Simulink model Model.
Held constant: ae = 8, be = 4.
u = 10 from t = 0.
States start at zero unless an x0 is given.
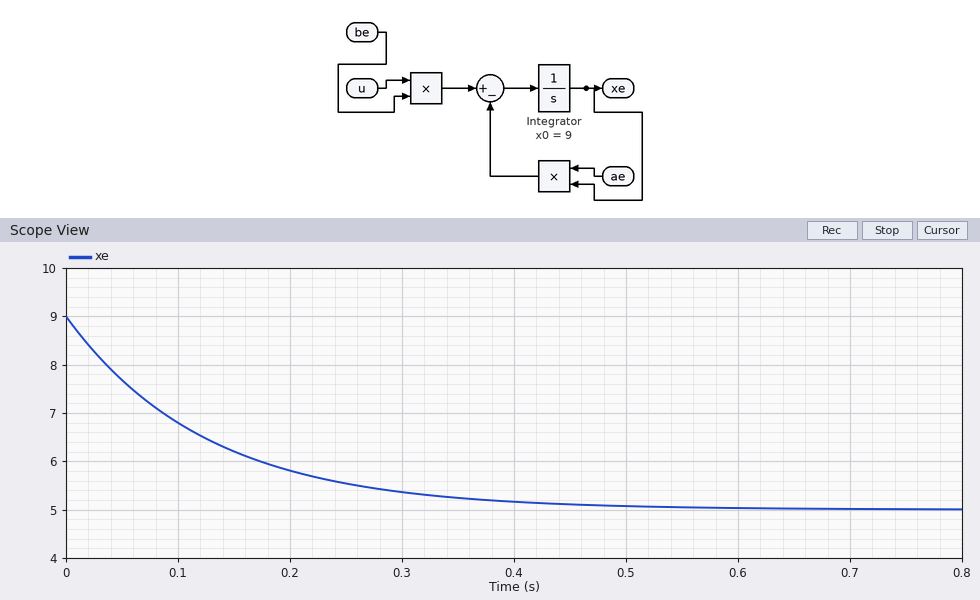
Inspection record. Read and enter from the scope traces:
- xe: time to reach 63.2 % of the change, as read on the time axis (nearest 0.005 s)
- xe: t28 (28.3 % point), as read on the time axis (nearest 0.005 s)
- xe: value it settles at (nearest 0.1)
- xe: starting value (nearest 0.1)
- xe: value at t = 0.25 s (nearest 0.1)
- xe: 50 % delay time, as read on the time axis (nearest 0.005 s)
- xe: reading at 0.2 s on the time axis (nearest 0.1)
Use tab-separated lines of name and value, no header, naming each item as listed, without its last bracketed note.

xe: time to reach 63.2 % of the change, as read on the time axis	0.125 s
xe: t28 (28.3 % point), as read on the time axis	0.040 s
xe: value it settles at	5.0
xe: starting value	9.0
xe: value at t = 0.25 s	5.5
xe: 50 % delay time, as read on the time axis	0.085 s
xe: reading at 0.2 s on the time axis	5.8
